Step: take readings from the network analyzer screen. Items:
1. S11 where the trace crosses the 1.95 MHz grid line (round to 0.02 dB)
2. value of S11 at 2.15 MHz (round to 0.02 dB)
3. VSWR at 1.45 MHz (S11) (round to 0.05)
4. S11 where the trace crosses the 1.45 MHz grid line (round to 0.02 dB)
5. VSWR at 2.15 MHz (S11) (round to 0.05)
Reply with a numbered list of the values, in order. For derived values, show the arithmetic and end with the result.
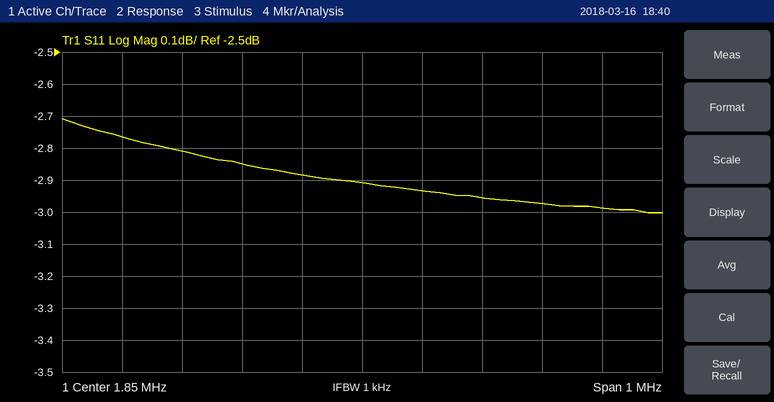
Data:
1. -2.94 dB
2. -2.98 dB
3. |Γ| = 10^(-2.76/20) = 0.7278; VSWR = (1 + 0.7278)/(1 − 0.7278) ≈ 6.35
4. -2.76 dB
5. |Γ| = 10^(-2.98/20) = 0.7096; VSWR = (1 + 0.7096)/(1 − 0.7096) ≈ 5.89, so 5.90 to the nearest 0.05
